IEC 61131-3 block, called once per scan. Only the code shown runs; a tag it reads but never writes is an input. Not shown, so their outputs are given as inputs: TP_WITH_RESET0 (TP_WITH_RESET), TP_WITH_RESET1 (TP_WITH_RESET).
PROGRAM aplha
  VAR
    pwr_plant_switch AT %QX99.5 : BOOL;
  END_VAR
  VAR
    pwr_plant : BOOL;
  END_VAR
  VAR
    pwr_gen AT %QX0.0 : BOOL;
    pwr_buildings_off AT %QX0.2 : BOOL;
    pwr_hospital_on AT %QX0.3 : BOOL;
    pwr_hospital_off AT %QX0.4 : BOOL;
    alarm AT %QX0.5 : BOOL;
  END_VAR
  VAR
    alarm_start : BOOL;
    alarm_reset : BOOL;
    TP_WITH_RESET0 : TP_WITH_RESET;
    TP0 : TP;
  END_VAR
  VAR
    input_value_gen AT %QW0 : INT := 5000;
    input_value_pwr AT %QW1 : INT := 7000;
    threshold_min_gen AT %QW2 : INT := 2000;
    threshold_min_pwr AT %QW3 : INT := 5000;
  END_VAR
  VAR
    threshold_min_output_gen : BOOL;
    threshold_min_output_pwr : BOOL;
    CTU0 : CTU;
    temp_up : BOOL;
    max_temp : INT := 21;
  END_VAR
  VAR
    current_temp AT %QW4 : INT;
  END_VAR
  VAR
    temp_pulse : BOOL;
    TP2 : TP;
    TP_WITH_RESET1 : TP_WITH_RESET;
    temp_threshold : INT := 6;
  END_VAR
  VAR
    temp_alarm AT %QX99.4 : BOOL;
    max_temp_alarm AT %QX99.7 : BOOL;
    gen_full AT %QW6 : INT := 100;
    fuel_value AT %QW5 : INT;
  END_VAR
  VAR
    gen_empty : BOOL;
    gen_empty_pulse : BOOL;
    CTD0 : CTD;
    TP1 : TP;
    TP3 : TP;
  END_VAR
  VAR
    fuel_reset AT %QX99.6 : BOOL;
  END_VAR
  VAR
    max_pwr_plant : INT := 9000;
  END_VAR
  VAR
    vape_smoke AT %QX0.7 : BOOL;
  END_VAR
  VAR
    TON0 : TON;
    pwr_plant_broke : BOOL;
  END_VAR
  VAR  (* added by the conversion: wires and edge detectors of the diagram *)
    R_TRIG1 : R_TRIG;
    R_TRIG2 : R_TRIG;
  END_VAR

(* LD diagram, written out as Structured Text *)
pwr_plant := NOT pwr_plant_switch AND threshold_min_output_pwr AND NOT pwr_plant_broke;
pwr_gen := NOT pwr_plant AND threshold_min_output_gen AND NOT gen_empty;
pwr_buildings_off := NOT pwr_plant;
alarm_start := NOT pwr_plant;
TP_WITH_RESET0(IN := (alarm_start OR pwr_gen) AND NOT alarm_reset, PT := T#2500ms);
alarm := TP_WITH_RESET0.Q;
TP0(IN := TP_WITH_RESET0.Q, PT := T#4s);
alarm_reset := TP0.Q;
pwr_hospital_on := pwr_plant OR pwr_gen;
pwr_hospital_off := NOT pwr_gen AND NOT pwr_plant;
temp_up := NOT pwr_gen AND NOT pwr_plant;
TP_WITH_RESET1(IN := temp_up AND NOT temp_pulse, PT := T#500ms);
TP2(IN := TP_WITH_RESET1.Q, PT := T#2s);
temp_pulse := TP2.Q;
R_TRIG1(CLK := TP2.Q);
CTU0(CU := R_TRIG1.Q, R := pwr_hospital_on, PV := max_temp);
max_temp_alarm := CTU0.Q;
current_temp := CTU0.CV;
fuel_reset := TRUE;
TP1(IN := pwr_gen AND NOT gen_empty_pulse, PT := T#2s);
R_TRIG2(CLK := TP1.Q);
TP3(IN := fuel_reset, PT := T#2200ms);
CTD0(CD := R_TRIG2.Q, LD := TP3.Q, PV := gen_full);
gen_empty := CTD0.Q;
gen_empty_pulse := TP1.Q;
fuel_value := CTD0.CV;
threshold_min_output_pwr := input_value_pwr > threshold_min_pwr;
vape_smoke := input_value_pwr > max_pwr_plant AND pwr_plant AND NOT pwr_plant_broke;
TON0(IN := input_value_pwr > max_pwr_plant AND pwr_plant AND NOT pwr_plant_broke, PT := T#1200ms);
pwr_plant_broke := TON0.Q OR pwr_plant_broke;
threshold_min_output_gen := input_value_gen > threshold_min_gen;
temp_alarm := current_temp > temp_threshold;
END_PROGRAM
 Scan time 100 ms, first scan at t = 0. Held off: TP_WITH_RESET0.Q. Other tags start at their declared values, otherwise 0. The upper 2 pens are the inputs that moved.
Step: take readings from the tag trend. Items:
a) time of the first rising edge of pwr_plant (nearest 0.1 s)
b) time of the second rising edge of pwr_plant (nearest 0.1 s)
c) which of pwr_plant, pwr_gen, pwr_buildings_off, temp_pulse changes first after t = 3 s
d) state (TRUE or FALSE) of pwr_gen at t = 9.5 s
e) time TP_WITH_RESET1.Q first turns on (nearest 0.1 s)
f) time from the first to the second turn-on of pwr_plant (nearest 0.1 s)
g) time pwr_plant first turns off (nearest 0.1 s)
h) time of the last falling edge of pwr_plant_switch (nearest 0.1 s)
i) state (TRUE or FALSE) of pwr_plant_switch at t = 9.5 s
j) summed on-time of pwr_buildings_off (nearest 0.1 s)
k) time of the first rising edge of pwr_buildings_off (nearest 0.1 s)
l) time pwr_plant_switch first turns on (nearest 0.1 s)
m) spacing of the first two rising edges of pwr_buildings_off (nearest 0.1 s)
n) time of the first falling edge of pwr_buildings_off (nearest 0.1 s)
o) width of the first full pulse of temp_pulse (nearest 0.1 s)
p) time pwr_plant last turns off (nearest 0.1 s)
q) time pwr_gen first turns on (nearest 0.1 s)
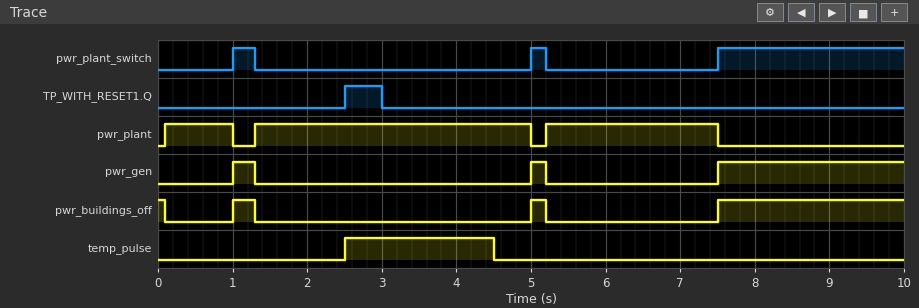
0.1 s
1.3 s
temp_pulse
TRUE
2.5 s
1.2 s
1.0 s
5.2 s
TRUE
3.1 s
1.0 s
1.0 s
4.0 s
0.1 s
2.0 s
7.5 s
1.0 s
